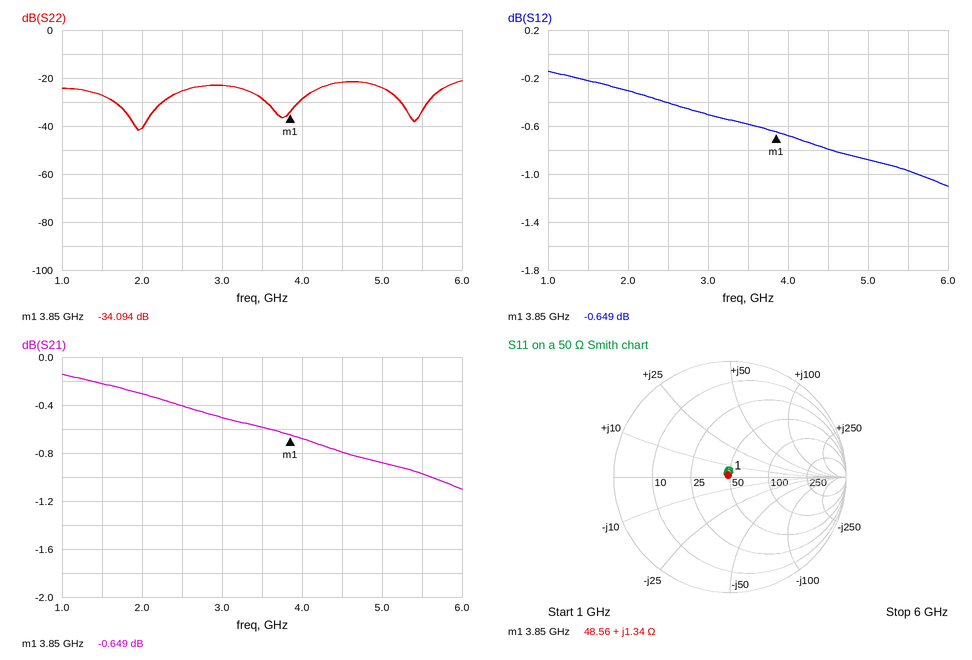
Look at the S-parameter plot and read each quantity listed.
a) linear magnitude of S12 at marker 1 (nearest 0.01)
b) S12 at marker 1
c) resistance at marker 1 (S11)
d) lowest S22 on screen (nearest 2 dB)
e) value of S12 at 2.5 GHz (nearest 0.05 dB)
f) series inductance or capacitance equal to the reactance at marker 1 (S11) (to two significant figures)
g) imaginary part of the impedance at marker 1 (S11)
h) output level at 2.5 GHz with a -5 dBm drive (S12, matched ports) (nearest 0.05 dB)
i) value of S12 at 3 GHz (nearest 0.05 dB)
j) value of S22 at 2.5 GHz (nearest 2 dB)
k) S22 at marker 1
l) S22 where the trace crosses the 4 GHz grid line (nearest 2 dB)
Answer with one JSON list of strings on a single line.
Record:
["0.93", "-0.649 dB", "48.56 Ω", "-42 dB", "-0.40 dB", "55 pH", "+1.34 Ω", "-5.40 dBm", "-0.50 dB", "-26 dB", "-34.094 dB", "-28 dB"]
